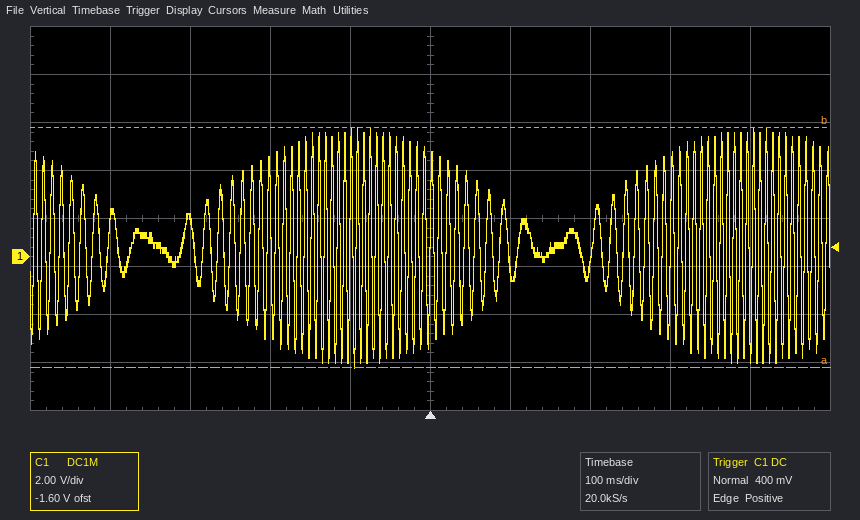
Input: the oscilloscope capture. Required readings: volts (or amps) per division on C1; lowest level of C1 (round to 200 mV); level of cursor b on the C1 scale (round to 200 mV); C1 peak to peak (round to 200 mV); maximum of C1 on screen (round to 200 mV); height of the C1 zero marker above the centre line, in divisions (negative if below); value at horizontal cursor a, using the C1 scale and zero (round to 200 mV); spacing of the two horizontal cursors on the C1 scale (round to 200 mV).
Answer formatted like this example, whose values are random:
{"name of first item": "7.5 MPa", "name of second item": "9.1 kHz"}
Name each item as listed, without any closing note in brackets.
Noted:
{"volts (or amps) per division on C1": "2 V", "lowest level of C1": "-4.6 V", "level of cursor b on the C1 scale": "5.4 V", "C1 peak to peak": "10.0 V", "maximum of C1 on screen": "5.4 V", "height of the C1 zero marker above the centre line, in divisions": "-0.8 div", "value at horizontal cursor a, using the C1 scale and zero": "-4.6 V", "spacing of the two horizontal cursors on the C1 scale": "10.0 V"}
